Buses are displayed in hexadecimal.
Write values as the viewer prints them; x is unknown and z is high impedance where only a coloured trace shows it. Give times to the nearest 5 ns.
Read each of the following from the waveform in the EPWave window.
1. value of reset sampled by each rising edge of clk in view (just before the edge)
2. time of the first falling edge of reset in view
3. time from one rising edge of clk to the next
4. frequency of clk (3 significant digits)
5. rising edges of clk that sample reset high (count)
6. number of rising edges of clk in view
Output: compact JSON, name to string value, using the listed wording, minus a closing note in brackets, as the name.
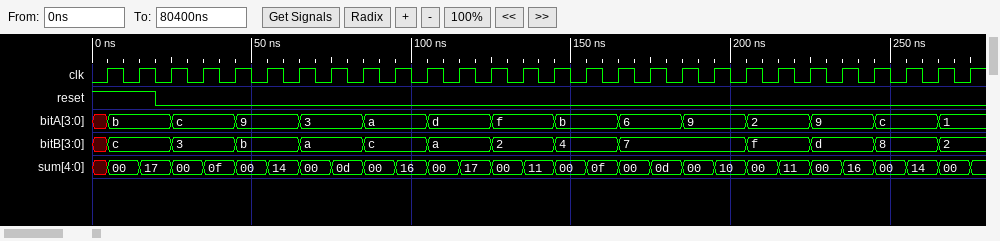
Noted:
{"value of reset sampled by each rising edge of clk in view": "1 1 0 0 0 0 0 0 0 0 0 0 0 0 0 0 0 0 0 0 0 0 0 0 0 0 0 0", "time of the first falling edge of reset in view": "20 ns", "time from one rising edge of clk to the next": "10 ns", "frequency of clk": "100 MHz", "rising edges of clk that sample reset high": "2", "number of rising edges of clk in view": "28"}
